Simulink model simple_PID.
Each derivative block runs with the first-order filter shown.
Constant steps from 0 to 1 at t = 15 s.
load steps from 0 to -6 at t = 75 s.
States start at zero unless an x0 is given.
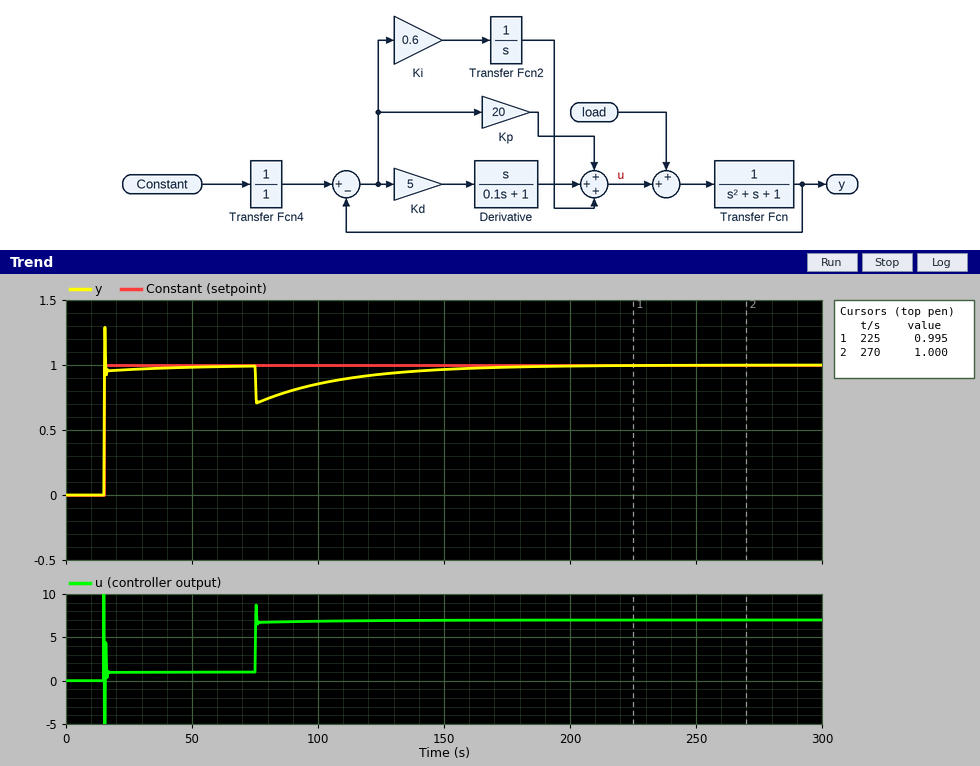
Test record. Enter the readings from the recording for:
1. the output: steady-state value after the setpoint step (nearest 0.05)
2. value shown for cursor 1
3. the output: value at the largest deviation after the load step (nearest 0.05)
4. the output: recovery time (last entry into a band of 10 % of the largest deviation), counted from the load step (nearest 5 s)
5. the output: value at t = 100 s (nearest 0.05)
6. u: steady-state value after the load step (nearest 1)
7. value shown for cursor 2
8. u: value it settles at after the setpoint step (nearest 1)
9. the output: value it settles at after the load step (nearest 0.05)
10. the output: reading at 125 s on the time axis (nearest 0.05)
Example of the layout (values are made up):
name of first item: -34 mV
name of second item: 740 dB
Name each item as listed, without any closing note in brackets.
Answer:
the output: steady-state value after the setpoint step: 1.00
value shown for cursor 1: 0.995
the output: value at the largest deviation after the load step: 0.70
the output: recovery time (last entry into a band of 10 % of the largest deviation), counted from the load step: 80 s
the output: value at t = 100 s: 0.85
u: steady-state value after the load step: 7
value shown for cursor 2: 1.000
u: value it settles at after the setpoint step: 1
the output: value it settles at after the load step: 1.00
the output: reading at 125 s on the time axis: 0.95
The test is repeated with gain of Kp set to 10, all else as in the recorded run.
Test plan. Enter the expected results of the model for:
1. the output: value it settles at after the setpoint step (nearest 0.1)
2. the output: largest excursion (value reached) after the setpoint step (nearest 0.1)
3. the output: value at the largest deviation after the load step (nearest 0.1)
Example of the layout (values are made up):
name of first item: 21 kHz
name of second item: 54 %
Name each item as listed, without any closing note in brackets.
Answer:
the output: value it settles at after the setpoint step: 1.0
the output: largest excursion (value reached) after the setpoint step: 1.1
the output: value at the largest deviation after the load step: 0.5
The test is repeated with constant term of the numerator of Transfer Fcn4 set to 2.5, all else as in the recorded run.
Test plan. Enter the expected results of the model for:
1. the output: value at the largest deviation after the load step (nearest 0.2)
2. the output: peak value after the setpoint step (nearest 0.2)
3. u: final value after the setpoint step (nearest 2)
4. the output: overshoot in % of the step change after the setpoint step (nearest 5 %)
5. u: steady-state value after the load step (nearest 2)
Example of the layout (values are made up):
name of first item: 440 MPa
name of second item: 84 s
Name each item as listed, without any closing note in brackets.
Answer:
the output: value at the largest deviation after the load step: 2.2
the output: peak value after the setpoint step: 3.2
u: final value after the setpoint step: 2
the output: overshoot in % of the step change after the setpoint step: 30 %
u: steady-state value after the load step: 8
